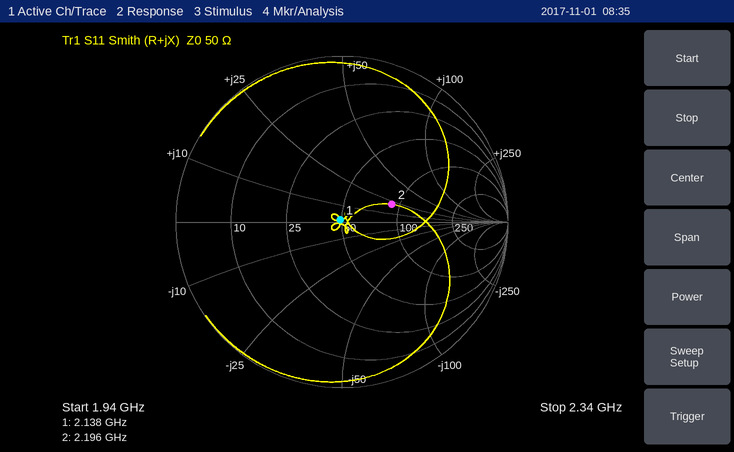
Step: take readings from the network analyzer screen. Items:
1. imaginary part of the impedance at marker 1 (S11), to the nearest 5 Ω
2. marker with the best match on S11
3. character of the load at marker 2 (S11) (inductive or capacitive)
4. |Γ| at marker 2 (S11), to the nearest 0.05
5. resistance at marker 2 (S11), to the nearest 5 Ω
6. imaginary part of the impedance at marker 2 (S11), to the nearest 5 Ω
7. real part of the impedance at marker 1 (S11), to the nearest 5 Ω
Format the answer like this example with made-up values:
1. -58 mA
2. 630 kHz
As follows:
1. 0 Ω
2. marker 1
3. inductive
4. 0.30
5. 90 Ω
6. +20 Ω
7. 50 Ω
